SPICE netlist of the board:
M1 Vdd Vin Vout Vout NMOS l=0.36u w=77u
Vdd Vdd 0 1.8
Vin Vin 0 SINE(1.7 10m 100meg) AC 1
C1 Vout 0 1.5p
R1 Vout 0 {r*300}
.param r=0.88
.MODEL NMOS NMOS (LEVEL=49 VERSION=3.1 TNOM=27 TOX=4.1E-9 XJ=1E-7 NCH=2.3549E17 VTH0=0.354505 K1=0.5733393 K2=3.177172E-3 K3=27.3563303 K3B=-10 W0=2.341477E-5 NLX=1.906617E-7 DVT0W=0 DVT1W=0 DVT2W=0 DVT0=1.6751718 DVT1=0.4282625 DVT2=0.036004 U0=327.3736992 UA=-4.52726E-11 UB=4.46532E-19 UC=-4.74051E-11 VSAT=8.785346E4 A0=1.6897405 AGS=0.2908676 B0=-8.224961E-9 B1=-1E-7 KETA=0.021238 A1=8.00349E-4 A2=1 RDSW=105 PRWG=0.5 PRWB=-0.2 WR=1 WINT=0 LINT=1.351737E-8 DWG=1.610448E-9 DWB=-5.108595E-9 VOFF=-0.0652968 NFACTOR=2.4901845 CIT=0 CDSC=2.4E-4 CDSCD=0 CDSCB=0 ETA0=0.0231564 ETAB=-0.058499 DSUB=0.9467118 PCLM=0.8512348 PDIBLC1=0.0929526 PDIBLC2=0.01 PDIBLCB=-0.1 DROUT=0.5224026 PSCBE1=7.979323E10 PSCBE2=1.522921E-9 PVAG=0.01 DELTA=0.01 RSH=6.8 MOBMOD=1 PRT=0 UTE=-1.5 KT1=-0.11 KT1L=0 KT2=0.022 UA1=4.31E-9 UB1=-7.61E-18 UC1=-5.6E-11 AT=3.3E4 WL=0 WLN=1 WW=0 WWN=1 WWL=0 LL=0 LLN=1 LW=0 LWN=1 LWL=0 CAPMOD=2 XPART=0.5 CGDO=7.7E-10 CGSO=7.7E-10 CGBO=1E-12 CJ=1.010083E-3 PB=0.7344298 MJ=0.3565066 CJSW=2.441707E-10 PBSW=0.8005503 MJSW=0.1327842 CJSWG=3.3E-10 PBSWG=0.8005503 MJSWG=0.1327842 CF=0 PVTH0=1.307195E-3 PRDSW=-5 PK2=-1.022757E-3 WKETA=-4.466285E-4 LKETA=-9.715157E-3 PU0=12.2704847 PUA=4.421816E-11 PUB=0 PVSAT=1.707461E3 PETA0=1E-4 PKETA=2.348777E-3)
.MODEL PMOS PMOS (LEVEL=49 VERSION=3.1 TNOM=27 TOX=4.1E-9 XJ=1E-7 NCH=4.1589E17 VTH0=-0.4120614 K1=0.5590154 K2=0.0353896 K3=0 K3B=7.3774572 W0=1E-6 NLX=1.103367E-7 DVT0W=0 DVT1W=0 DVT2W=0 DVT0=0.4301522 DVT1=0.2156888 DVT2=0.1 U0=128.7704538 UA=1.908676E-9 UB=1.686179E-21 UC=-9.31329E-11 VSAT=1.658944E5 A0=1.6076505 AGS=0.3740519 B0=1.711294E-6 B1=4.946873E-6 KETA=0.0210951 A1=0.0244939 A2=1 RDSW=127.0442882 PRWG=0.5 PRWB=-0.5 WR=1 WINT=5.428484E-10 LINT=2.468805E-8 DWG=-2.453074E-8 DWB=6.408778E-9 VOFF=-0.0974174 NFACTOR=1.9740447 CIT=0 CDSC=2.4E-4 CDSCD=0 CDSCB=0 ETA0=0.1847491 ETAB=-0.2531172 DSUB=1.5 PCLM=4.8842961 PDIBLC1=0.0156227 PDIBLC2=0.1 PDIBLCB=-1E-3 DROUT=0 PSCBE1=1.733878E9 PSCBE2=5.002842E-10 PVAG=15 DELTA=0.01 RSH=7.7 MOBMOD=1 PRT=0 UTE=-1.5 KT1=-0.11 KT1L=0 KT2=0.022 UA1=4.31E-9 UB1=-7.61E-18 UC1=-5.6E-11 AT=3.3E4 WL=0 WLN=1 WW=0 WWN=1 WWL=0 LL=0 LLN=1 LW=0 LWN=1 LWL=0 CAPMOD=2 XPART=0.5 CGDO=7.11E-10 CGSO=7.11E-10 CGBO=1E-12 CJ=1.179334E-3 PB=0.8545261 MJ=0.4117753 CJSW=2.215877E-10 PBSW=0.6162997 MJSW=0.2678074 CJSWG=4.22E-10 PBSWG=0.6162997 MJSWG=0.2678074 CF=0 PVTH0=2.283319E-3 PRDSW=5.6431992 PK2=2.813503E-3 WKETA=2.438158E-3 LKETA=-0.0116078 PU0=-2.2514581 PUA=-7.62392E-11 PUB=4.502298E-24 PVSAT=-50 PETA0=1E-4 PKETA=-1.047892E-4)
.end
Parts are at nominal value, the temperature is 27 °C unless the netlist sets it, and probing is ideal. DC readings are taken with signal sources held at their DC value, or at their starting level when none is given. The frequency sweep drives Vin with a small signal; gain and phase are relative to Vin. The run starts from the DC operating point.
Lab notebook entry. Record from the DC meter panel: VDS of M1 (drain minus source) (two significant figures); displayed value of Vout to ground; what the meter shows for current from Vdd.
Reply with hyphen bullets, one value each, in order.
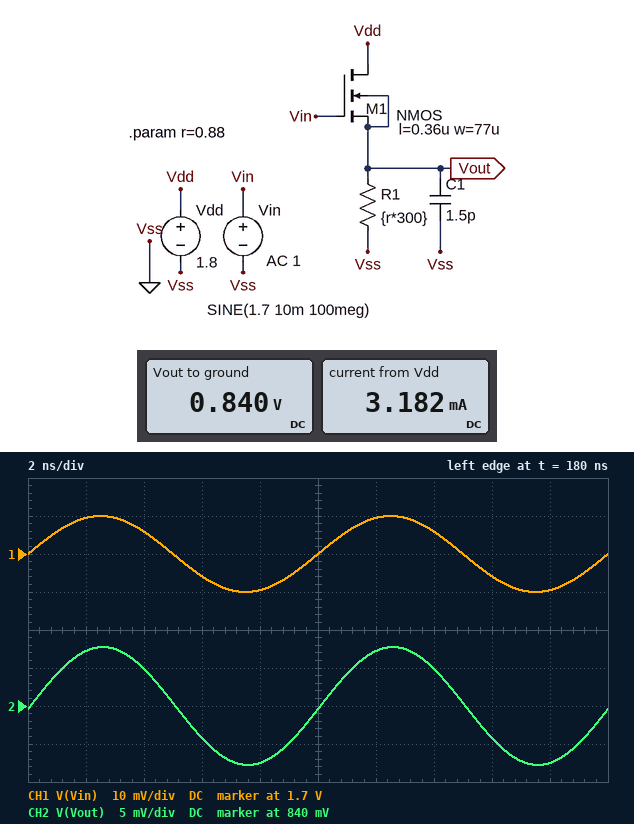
- 960 mV
- 0.840 V
- 3.182 mA
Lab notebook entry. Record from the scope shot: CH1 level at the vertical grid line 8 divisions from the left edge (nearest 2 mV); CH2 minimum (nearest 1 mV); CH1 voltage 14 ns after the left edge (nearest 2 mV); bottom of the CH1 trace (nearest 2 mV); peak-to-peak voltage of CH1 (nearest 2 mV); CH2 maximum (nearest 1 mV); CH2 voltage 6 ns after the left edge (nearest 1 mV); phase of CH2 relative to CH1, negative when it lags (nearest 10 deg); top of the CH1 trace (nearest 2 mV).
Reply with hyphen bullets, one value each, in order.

- 1.694 V
- 832 mV
- 1.706 V
- 1.690 V
- 20 mV
- 848 mV
- 836 mV
- 0 deg
- 1.710 V
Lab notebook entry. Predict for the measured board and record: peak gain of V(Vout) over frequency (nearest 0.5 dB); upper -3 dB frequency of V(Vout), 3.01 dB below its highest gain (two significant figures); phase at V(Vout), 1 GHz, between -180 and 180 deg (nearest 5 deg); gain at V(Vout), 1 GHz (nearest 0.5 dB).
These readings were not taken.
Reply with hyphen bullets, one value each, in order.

- -2.0 dB
- 1.7 GHz
- -25 deg
- -3.5 dB
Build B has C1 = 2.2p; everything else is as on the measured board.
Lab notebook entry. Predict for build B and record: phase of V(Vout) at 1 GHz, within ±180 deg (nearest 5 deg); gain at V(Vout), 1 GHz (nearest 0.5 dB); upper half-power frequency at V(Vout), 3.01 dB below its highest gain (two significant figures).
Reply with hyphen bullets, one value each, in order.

- -35 deg
- -4.5 dB
- 1.2 GHz
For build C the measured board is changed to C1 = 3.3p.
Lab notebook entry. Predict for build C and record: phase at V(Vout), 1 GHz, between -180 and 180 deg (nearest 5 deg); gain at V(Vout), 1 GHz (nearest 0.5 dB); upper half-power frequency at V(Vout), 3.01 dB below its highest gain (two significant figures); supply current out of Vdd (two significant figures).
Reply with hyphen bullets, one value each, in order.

- -45 deg
- -6.0 dB
- 820 MHz
- 3.2 mA
